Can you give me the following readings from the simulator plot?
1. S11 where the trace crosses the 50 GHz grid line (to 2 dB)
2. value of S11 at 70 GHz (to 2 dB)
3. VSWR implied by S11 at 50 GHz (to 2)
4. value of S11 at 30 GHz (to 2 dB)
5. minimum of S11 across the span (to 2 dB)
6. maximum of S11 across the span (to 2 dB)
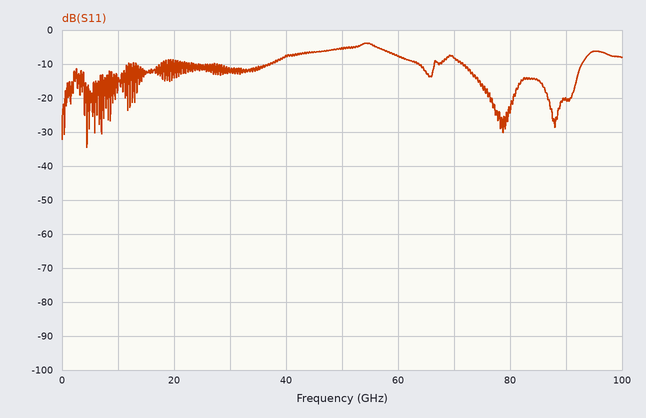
-6 dB
-8 dB
4
-12 dB
-34 dB
-4 dB
